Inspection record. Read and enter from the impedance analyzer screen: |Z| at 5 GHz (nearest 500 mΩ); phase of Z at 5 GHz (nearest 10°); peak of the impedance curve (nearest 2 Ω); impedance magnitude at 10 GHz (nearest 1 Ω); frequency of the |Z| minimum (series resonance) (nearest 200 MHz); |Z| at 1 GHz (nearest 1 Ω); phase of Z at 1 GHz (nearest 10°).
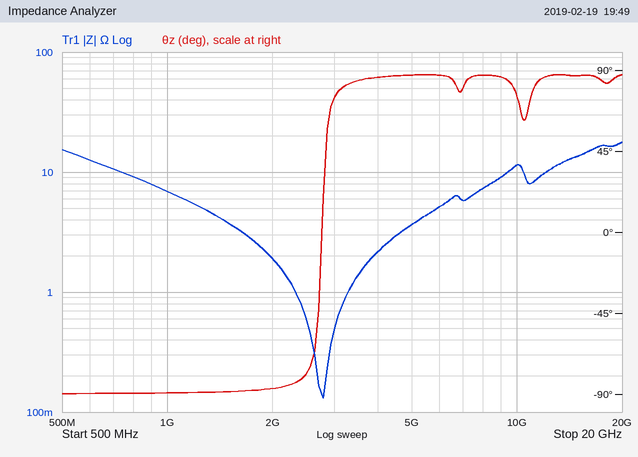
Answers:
3.5 Ω
90°
18 Ω
11 Ω
2.8 GHz
7 Ω
-90°
